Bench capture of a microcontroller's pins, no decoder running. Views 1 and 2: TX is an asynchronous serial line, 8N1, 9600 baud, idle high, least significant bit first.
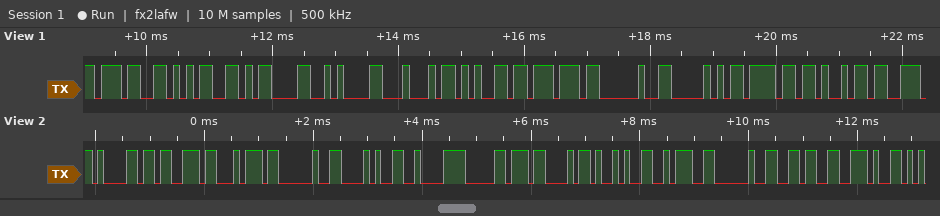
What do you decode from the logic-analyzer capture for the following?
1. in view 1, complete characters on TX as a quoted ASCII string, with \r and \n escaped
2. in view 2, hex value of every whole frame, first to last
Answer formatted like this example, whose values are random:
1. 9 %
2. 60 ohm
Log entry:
1. "75\r\nDew Poi"
2. 0x61 0x73 0x74 0x20 0x28 0xC2 0xB0 0x43 0x29 0x3A 0x20 0x36 0x2E
